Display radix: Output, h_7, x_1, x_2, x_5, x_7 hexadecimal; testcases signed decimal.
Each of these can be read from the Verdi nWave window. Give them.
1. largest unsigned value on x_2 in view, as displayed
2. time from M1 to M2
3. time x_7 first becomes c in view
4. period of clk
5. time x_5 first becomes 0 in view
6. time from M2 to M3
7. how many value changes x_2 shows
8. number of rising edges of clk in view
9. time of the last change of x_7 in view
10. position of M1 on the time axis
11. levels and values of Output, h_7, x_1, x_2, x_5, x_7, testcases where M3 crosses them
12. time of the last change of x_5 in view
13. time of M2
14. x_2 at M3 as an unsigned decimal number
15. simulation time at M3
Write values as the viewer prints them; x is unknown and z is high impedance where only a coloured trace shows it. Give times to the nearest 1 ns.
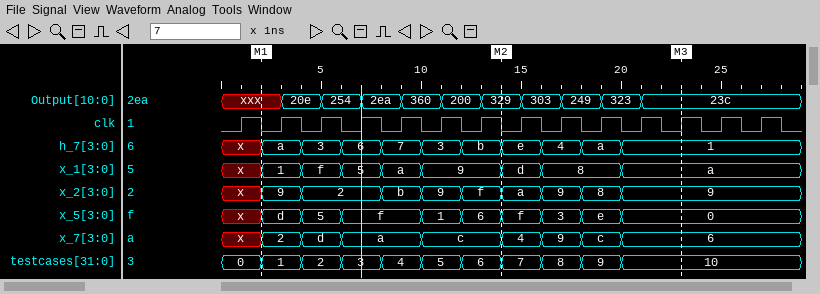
f
12 ns
10 ns
2 ns
20 ns
9 ns
9
14
20 ns
2 ns
Output=23c, h_7=1, x_1=a, x_2=9, x_5=0, x_7=6, testcases=10
20 ns
14 ns
9
23 ns
